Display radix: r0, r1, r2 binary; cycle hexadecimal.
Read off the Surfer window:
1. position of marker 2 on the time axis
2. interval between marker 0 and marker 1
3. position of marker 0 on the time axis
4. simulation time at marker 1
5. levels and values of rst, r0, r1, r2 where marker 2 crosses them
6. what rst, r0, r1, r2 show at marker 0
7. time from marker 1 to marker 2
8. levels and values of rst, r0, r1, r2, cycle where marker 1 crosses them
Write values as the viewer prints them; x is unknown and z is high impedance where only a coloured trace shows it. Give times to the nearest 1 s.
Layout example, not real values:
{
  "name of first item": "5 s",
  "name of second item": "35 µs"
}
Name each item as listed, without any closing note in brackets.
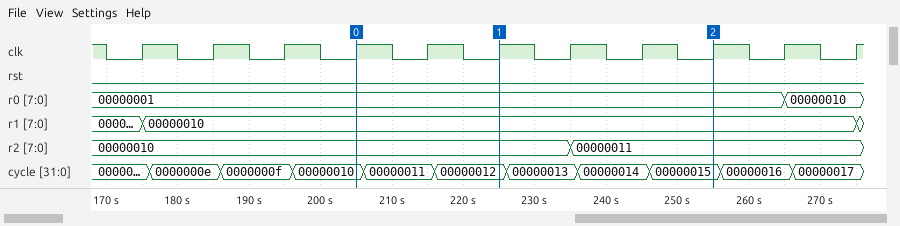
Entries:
{
  "position of marker 2 on the time axis": "255 s",
  "interval between marker 0 and marker 1": "20 s",
  "position of marker 0 on the time axis": "205 s",
  "simulation time at marker 1": "225 s",
  "levels and values of rst, r0, r1, r2 where marker 2 crosses them": "rst=0, r0=00000001, r1=00000010, r2=00000011",
  "what rst, r0, r1, r2 show at marker 0": "rst=0, r0=00000001, r1=00000010, r2=00000010",
  "time from marker 1 to marker 2": "30 s",
  "levels and values of rst, r0, r1, r2, cycle where marker 1 crosses them": "rst=0, r0=00000001, r1=00000010, r2=00000010, cycle=00000012"
}
